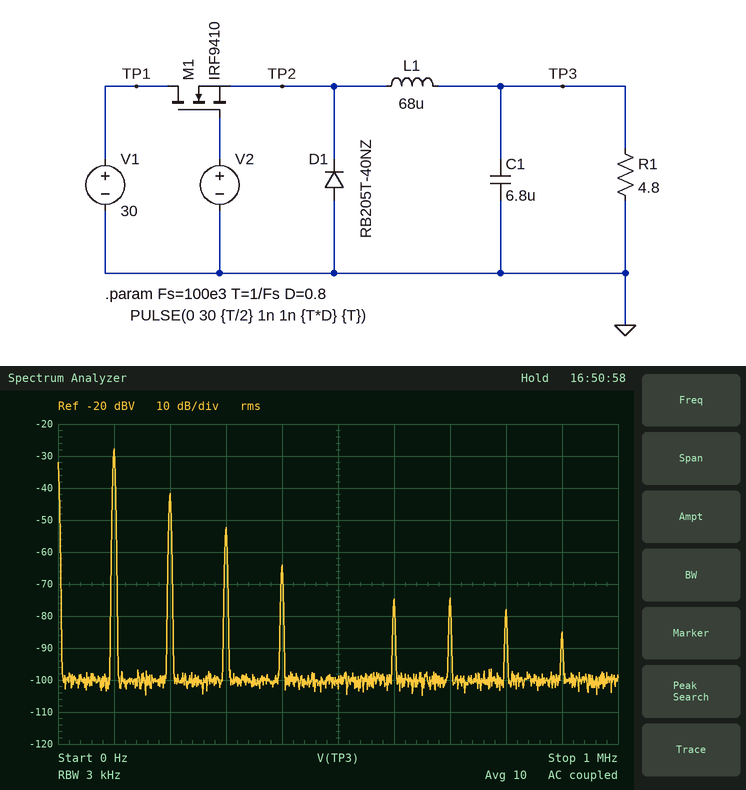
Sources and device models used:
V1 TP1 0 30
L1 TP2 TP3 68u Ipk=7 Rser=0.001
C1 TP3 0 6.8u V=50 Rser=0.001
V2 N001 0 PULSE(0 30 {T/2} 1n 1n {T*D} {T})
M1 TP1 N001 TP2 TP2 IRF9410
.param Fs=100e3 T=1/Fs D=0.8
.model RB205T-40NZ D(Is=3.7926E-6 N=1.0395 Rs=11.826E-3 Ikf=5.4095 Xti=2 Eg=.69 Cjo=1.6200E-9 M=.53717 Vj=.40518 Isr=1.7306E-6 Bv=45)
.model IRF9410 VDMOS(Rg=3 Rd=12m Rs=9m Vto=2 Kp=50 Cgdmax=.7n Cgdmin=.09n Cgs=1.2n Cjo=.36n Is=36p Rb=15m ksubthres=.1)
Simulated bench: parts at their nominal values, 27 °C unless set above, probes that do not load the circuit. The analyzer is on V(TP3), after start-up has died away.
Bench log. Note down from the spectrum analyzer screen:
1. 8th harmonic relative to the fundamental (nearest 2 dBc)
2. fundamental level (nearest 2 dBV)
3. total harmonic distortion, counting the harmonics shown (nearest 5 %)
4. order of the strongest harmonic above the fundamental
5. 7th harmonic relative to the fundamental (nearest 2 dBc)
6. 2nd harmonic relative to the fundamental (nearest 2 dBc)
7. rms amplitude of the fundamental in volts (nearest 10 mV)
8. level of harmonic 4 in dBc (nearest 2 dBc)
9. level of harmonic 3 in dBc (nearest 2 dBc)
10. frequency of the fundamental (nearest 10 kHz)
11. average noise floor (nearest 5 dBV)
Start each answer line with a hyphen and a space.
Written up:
- -50 dBc
- -28 dBV
- 20 %
- 2
- -46 dBc
- -14 dBc
- 40 mV
- -36 dBc
- -24 dBc
- 100 kHz
- -100 dBV
